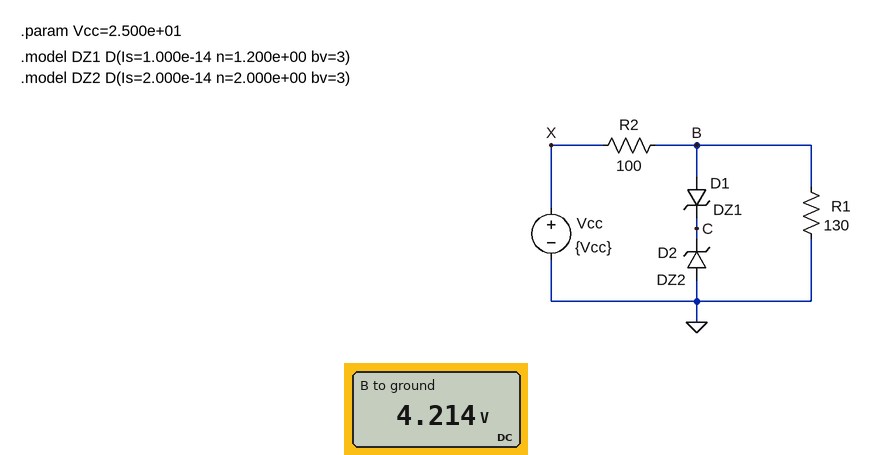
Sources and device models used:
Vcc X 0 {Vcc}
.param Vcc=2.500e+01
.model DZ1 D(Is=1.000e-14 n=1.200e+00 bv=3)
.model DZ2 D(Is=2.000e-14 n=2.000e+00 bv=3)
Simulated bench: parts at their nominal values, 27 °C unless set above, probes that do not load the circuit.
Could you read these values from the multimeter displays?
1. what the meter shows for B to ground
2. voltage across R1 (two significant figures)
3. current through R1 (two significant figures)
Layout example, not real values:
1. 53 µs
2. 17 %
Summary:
1. 4.214 V
2. 4.2 V
3. 32 mA
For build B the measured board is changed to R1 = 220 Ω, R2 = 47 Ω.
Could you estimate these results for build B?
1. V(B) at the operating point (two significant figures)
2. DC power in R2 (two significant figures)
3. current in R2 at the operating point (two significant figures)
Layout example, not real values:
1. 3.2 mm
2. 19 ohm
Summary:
1. 4.3 V
2. 9.1 W
3. 440 mA
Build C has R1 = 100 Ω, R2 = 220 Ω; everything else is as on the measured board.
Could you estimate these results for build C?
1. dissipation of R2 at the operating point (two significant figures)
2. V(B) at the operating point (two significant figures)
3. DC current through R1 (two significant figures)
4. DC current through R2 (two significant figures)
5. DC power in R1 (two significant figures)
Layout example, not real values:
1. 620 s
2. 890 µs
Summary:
1. 2.0 W
2. 4.1 V
3. 41 mA
4. 95 mA
5. 170 mW
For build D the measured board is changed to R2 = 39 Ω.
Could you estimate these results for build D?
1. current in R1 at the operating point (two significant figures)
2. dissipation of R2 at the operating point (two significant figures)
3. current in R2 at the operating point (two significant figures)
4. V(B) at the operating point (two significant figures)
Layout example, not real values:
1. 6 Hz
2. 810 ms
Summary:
1. 33 mA
2. 11 W
3. 530 mA
4. 4.3 V
